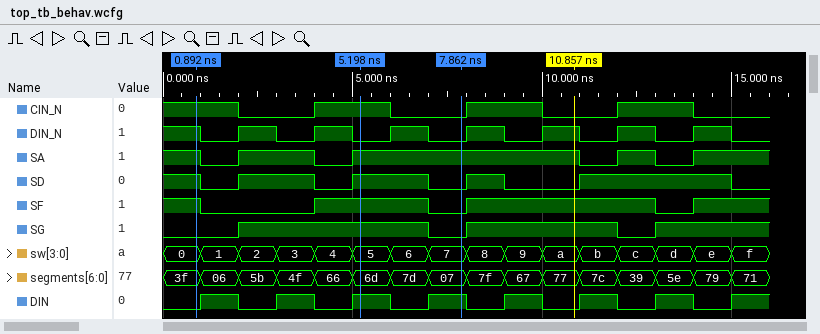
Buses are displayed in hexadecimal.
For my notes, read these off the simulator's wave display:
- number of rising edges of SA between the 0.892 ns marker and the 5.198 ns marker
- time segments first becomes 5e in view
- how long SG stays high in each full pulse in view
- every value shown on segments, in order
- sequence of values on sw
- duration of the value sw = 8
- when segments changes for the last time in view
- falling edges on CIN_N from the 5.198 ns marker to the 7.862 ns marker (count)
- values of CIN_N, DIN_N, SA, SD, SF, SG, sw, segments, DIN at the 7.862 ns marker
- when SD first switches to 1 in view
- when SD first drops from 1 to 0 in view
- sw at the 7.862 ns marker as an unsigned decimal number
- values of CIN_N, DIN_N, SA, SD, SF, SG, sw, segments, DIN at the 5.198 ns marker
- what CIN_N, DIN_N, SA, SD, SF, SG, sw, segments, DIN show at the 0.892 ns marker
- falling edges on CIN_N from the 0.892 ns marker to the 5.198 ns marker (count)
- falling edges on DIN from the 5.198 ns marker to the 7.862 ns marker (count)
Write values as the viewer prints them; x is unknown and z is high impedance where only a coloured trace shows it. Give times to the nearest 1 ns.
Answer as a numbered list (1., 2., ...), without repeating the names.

1. 2
2. 13 ns
3. 5 ns, 4 ns
4. 3f, 06, 5b, 4f, 66, 6d, 7d, 07, 7f, 67, 77, 7c, 39, 5e, 79, 71
5. 0, 1, 2, 3, 4, 5, 6, 7, 8, 9, a, b, c, d, e, f
6. 1 ns
7. 15 ns
8. 1
9. CIN_N=0, DIN_N=0, SA=1, SD=0, SF=0, SG=0, sw=7, segments=07, DIN=1
10. 2 ns
11. 1 ns
12. 7
13. CIN_N=1, DIN_N=0, SA=1, SD=1, SF=1, SG=1, sw=5, segments=6d, DIN=1
14. CIN_N=1, DIN_N=1, SA=1, SD=1, SF=1, SG=0, sw=0, segments=3f, DIN=0
15. 1
16. 1
